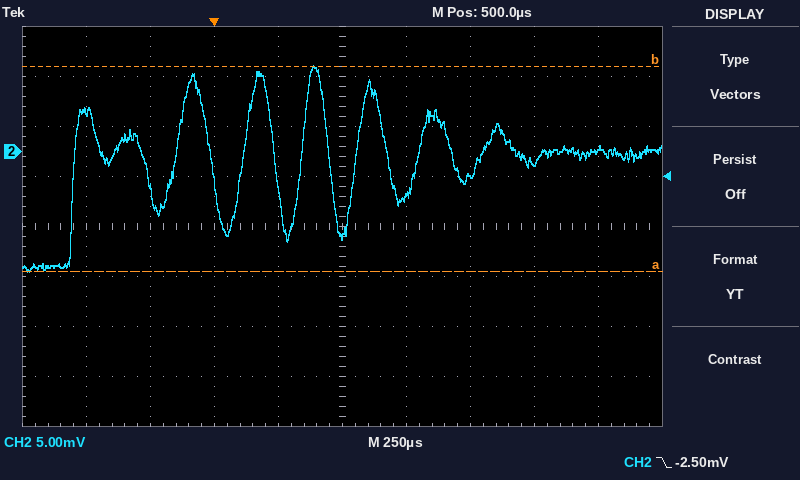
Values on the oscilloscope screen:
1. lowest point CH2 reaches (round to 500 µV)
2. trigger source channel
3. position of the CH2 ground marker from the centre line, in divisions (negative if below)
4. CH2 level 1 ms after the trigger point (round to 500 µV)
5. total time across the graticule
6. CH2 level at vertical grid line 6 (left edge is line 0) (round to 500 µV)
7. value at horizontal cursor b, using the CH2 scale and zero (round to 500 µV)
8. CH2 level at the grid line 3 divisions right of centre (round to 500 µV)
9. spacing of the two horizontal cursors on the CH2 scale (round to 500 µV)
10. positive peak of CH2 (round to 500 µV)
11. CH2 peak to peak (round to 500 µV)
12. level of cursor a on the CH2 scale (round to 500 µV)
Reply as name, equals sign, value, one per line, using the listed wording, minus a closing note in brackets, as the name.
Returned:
lowest point CH2 reaches = -12.0 mV
trigger source channel = CH2
position of the CH2 ground marker from the centre line, in divisions = +1.5 div
CH2 level 1 ms after the trigger point = -2.5 mV
total time across the graticule = 2.5 ms
CH2 level at vertical grid line 6 (left edge is line 0) = -4.5 mV
value at horizontal cursor b, using the CH2 scale and zero = 8.5 mV
CH2 level at the grid line 3 divisions right of centre = -1.0 mV
spacing of the two horizontal cursors on the CH2 scale = 20.5 mV
positive peak of CH2 = 8.5 mV
CH2 peak to peak = 20.5 mV
level of cursor a on the CH2 scale = -12.0 mV
